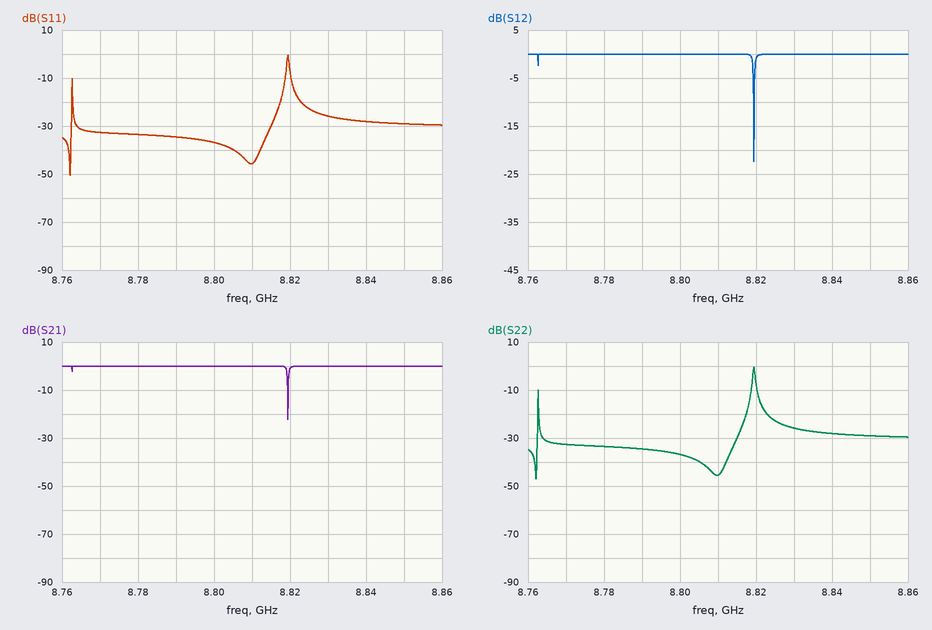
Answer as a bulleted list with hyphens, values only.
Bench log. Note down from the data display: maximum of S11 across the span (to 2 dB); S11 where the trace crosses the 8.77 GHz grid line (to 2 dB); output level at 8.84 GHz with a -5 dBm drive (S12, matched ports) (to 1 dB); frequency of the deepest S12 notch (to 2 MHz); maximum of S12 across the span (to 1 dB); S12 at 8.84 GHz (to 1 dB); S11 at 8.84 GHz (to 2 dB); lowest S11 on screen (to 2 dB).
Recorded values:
- 0 dB
- -32 dB
- -5 dBm
- 8.820 GHz
- 0 dB
- 0 dB
- -28 dB
- -50 dB
